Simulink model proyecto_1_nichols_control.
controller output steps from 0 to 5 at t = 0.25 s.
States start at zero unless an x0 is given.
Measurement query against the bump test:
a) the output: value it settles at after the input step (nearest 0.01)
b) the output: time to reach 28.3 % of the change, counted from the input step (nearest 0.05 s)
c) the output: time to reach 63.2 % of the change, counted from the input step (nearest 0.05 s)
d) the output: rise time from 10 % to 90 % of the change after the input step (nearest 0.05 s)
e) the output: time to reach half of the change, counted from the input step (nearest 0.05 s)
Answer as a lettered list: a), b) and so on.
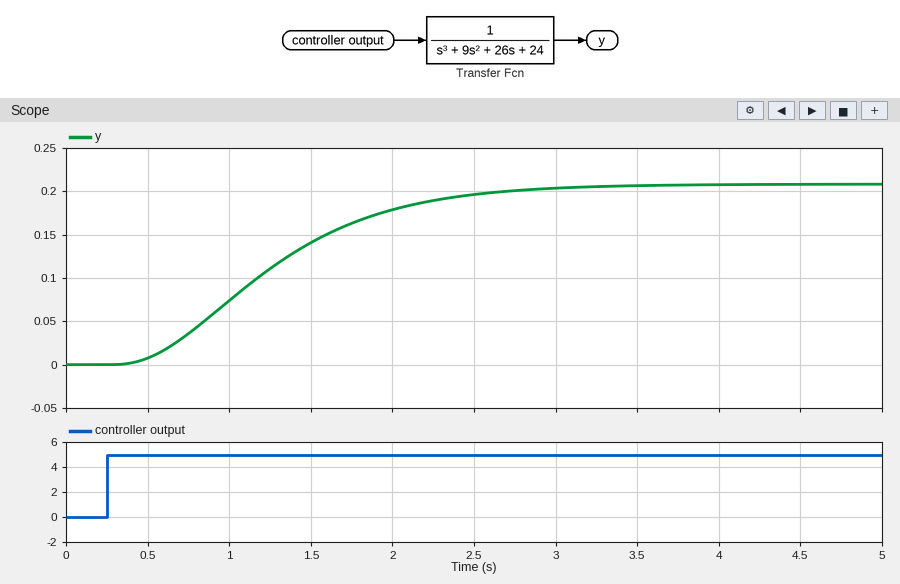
a) 0.21
b) 0.65 s
c) 1.15 s
d) 1.55 s
e) 0.95 s
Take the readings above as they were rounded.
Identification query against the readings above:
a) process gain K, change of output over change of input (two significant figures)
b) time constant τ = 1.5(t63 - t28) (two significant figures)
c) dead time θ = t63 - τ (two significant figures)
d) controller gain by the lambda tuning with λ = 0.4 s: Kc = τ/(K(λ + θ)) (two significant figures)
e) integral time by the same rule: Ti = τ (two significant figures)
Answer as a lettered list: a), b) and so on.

a) 0.042
b) 0.75 s
c) 0.40 s
d) 22
e) 0.75 s
